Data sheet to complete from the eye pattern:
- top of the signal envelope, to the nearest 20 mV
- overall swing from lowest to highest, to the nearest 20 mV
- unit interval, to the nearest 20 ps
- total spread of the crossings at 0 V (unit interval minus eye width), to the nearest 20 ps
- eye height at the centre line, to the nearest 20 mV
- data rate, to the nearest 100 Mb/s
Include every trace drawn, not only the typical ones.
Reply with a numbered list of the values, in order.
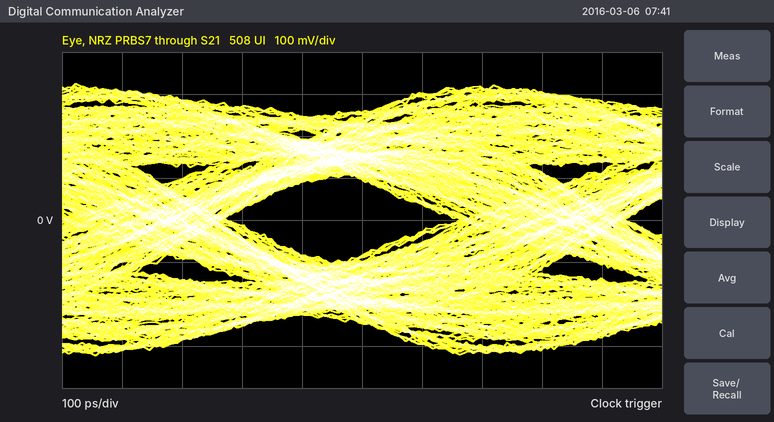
1. 320 mV
2. 640 mV
3. 660 ps
4. 280 ps
5. 180 mV
6. 1.5 Gb/s
